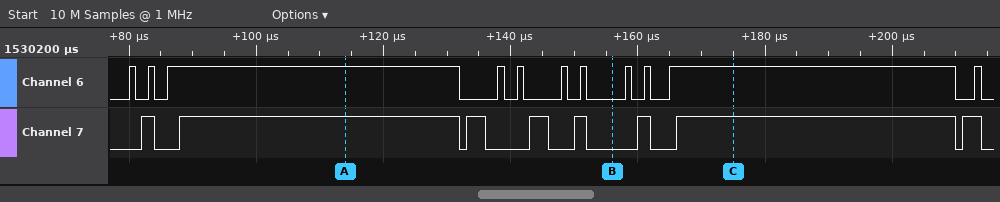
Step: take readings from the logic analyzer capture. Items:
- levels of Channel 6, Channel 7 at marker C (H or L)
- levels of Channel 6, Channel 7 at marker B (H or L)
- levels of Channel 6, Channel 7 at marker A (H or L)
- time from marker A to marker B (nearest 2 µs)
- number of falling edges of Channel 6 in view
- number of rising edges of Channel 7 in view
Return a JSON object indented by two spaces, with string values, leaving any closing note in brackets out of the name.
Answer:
{
  "levels of Channel 6, Channel 7 at marker C": "Channel 6=H, Channel 7=H",
  "levels of Channel 6, Channel 7 at marker B": "Channel 6=L, Channel 7=L",
  "levels of Channel 6, Channel 7 at marker A": "Channel 6=H, Channel 7=H",
  "time from marker A to marker B": "42 µs",
  "number of falling edges of Channel 6 in view": "11",
  "number of rising edges of Channel 7 in view": "8"
}
